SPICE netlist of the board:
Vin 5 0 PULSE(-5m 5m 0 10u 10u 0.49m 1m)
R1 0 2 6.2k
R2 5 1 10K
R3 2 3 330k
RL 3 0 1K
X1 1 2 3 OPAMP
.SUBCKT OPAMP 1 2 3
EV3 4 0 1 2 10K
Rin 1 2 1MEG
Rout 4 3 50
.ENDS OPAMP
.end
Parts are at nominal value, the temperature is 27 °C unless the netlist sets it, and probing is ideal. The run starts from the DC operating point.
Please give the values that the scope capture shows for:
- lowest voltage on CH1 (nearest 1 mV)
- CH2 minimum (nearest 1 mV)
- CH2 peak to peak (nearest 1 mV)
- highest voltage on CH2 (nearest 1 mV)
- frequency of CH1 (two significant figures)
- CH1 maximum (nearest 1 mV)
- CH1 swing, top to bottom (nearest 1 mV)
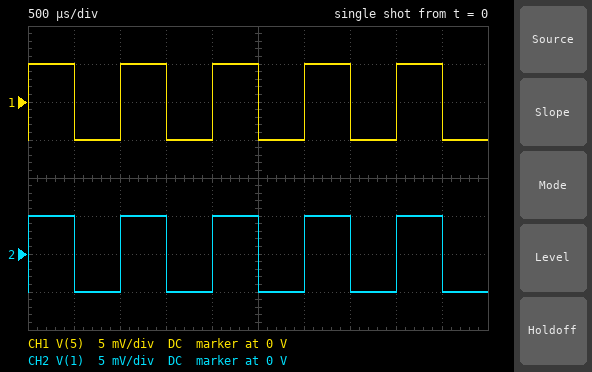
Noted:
-5 mV
-5 mV
10 mV
5 mV
1.0 kHz
5 mV
10 mV
